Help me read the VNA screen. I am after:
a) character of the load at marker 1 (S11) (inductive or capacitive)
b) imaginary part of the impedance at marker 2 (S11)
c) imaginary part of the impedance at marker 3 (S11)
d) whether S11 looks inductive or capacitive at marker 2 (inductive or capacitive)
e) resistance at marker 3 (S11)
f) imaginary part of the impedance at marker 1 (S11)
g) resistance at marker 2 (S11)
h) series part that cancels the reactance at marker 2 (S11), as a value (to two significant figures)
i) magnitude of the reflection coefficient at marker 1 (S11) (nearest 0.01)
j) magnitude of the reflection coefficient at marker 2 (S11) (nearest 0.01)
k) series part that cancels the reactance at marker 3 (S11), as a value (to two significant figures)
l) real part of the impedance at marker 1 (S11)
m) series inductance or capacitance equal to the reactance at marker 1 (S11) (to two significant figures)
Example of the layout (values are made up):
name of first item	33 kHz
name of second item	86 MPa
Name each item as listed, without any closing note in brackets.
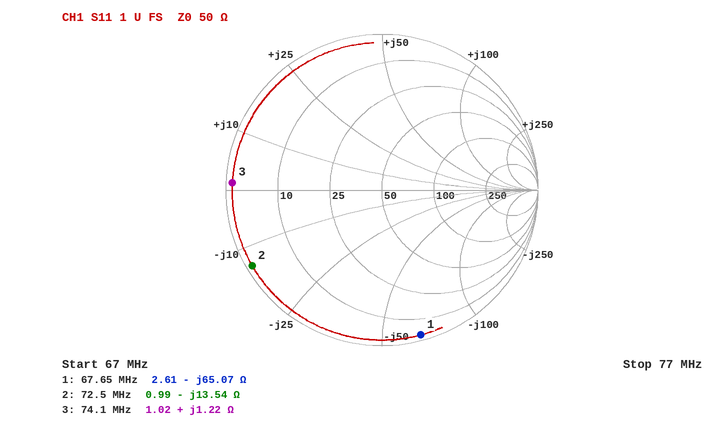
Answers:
character of the load at marker 1 (S11)	capacitive
imaginary part of the impedance at marker 2	-13.54 Ω
imaginary part of the impedance at marker 3	+1.22 Ω
whether S11 looks inductive or capacitive at marker 2	capacitive
resistance at marker 3	1.02 Ω
imaginary part of the impedance at marker 1	-65.07 Ω
resistance at marker 2	0.99 Ω
series part that cancels the reactance at marker 2 (S11), as a value	30 nH
magnitude of the reflection coefficient at marker 1 (S11)	0.96
magnitude of the reflection coefficient at marker 2 (S11)	0.96
series part that cancels the reactance at marker 3 (S11), as a value	1.8 nF
real part of the impedance at marker 1	2.61 Ω
series inductance or capacitance equal to the reactance at marker 1 (S11)	36 pF
